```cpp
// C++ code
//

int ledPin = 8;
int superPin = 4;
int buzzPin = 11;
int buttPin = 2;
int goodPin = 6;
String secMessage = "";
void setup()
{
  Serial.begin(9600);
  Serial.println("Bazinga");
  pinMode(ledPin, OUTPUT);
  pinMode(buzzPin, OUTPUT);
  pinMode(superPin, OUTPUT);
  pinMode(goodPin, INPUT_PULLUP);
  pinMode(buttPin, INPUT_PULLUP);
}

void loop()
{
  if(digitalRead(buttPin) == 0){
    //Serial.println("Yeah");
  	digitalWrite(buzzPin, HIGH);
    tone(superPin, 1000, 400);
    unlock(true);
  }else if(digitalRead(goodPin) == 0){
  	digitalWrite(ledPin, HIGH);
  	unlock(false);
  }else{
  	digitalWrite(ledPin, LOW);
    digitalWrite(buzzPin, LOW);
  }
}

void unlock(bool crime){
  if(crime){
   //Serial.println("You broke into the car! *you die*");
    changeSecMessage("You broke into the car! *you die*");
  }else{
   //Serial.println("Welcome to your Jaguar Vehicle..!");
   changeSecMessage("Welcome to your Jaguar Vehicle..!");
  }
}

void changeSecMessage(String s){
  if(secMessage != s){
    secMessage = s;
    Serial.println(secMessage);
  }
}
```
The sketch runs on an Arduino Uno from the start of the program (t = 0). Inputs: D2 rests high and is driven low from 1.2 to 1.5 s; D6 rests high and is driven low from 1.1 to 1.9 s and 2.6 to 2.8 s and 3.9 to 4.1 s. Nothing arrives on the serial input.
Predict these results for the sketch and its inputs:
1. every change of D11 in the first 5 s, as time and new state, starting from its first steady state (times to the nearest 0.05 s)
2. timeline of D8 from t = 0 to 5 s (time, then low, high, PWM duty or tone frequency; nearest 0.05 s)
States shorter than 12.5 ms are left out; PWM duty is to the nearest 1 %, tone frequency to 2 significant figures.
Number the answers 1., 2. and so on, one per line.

1. 0 s low; 1.2 s high; 1.9 s low
2. 0 s low; 1.1 s high; 1.9 s low; 2.6 s high; 2.8 s low; 3.9 s high; 4.1 s low
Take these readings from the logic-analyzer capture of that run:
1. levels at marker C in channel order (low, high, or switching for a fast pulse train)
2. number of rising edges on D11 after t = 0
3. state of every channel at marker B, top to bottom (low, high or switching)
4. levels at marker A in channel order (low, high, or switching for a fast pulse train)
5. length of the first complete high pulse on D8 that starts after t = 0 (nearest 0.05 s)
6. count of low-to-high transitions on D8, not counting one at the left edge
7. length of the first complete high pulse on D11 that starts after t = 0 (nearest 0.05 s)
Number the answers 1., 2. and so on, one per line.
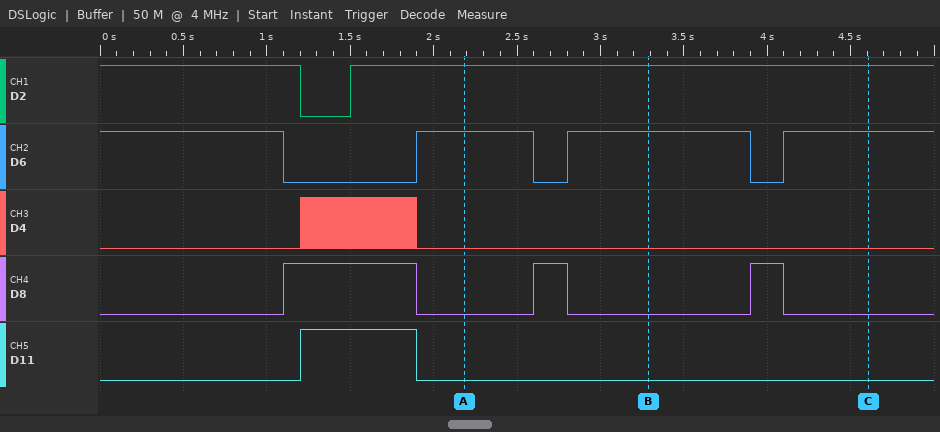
1. D2 high, D6 high, D4 low, D8 low, D11 low
2. 1
3. D2 high, D6 high, D4 low, D8 low, D11 low
4. D2 high, D6 high, D4 low, D8 low, D11 low
5. 0.80 s
6. 3
7. 0.70 s
